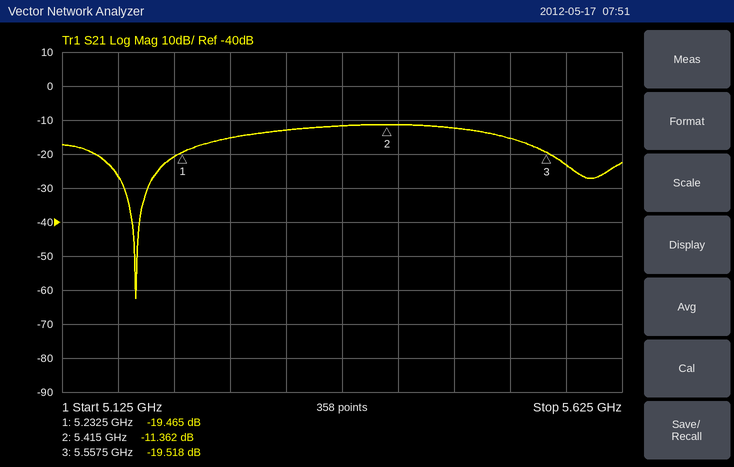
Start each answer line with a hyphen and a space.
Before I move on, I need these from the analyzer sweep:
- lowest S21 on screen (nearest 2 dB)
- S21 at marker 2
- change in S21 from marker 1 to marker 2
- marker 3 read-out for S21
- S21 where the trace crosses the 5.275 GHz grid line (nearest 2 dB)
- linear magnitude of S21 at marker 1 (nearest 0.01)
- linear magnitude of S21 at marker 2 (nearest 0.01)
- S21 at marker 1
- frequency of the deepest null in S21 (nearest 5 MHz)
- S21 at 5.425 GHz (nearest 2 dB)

- -62 dB
- -11.362 dB
- 8.103 dB
- -19.518 dB
- -16 dB
- 0.11
- 0.27
- -19.465 dB
- 5.190 GHz
- -12 dB
